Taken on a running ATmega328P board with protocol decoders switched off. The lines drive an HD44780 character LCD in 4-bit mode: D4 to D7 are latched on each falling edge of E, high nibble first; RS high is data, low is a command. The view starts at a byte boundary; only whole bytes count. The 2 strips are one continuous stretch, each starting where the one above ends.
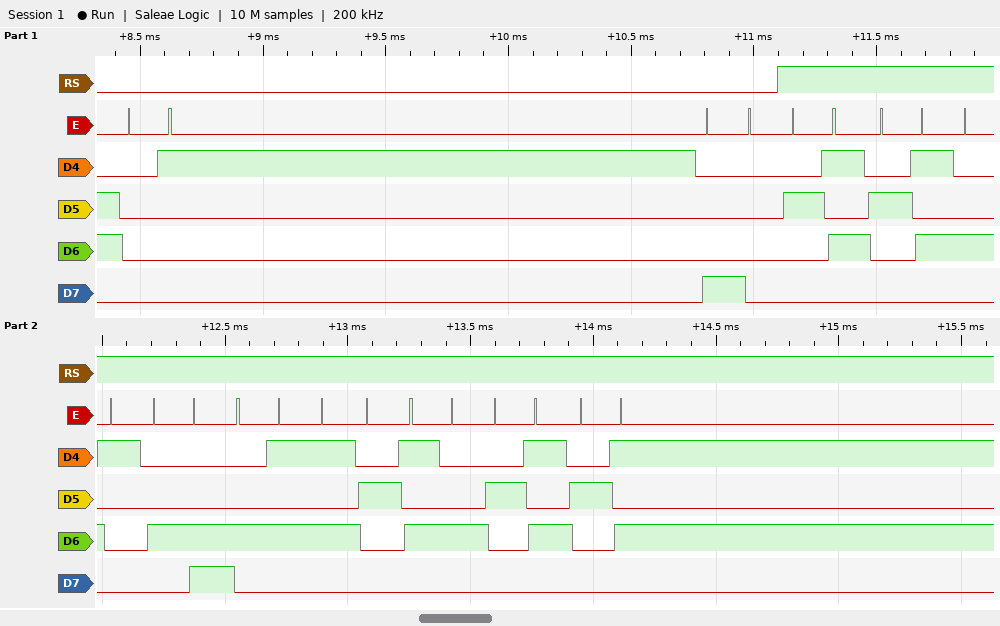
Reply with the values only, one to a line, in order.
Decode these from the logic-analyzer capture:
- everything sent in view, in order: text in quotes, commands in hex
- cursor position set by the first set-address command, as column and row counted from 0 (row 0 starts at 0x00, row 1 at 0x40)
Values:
0x01 0x80 "%%ALERT%%"
column 0, row 0
